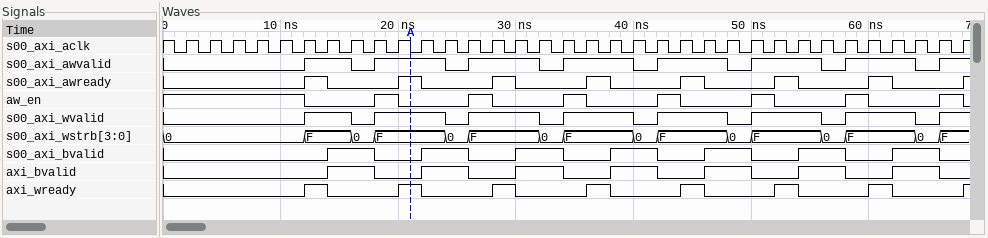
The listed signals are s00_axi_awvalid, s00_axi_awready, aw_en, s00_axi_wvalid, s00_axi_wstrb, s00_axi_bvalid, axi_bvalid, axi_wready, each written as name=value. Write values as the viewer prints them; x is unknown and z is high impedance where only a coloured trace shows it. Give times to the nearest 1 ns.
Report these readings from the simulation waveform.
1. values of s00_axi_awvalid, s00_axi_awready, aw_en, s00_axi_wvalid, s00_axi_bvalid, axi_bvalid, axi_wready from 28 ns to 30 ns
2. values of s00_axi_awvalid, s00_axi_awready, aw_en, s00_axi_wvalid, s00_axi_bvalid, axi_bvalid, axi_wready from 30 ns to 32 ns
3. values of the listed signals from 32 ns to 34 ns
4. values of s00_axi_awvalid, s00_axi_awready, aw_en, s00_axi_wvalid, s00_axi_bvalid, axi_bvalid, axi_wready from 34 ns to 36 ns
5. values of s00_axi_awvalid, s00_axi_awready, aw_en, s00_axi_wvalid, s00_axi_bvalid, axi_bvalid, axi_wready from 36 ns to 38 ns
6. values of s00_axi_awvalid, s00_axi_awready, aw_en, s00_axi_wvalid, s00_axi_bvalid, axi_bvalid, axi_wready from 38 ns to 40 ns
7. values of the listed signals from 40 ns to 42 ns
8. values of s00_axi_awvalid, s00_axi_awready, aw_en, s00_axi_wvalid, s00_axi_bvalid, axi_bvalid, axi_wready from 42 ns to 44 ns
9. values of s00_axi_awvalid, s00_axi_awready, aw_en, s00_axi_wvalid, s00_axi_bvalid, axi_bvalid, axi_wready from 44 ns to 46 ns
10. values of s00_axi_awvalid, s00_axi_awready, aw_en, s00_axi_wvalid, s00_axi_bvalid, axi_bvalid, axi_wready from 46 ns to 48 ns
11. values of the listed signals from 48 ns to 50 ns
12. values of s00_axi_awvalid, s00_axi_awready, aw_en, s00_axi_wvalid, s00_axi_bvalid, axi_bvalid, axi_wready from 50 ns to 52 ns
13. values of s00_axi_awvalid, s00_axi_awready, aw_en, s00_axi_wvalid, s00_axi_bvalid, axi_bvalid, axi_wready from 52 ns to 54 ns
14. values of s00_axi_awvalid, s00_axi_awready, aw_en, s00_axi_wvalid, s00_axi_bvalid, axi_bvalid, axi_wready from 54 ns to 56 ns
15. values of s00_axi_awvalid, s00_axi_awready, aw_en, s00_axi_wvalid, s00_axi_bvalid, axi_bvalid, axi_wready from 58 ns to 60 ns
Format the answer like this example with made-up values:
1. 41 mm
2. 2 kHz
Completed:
1. s00_axi_awvalid=1, s00_axi_awready=1, aw_en=0, s00_axi_wvalid=1, s00_axi_bvalid=0, axi_bvalid=0, axi_wready=1
2. s00_axi_awvalid=1, s00_axi_awready=0, aw_en=0, s00_axi_wvalid=1, s00_axi_bvalid=1, axi_bvalid=1, axi_wready=0
3. s00_axi_awvalid=0, s00_axi_awready=0, aw_en=0, s00_axi_wvalid=0, s00_axi_wstrb=0, s00_axi_bvalid=1, axi_bvalid=1, axi_wready=0
4. s00_axi_awvalid=1, s00_axi_awready=0, aw_en=1, s00_axi_wvalid=1, s00_axi_bvalid=0, axi_bvalid=0, axi_wready=0
5. s00_axi_awvalid=1, s00_axi_awready=1, aw_en=0, s00_axi_wvalid=1, s00_axi_bvalid=0, axi_bvalid=0, axi_wready=1
6. s00_axi_awvalid=1, s00_axi_awready=0, aw_en=0, s00_axi_wvalid=1, s00_axi_bvalid=1, axi_bvalid=1, axi_wready=0
7. s00_axi_awvalid=0, s00_axi_awready=0, aw_en=0, s00_axi_wvalid=0, s00_axi_wstrb=0, s00_axi_bvalid=1, axi_bvalid=1, axi_wready=0
8. s00_axi_awvalid=1, s00_axi_awready=0, aw_en=1, s00_axi_wvalid=1, s00_axi_bvalid=0, axi_bvalid=0, axi_wready=0
9. s00_axi_awvalid=1, s00_axi_awready=1, aw_en=0, s00_axi_wvalid=1, s00_axi_bvalid=0, axi_bvalid=0, axi_wready=1
10. s00_axi_awvalid=1, s00_axi_awready=0, aw_en=0, s00_axi_wvalid=1, s00_axi_bvalid=1, axi_bvalid=1, axi_wready=0
11. s00_axi_awvalid=0, s00_axi_awready=0, aw_en=0, s00_axi_wvalid=0, s00_axi_wstrb=0, s00_axi_bvalid=1, axi_bvalid=1, axi_wready=0
12. s00_axi_awvalid=1, s00_axi_awready=0, aw_en=1, s00_axi_wvalid=1, s00_axi_bvalid=0, axi_bvalid=0, axi_wready=0
13. s00_axi_awvalid=1, s00_axi_awready=1, aw_en=0, s00_axi_wvalid=1, s00_axi_bvalid=0, axi_bvalid=0, axi_wready=1
14. s00_axi_awvalid=1, s00_axi_awready=0, aw_en=0, s00_axi_wvalid=1, s00_axi_bvalid=1, axi_bvalid=1, axi_wready=0
15. s00_axi_awvalid=1, s00_axi_awready=0, aw_en=1, s00_axi_wvalid=1, s00_axi_bvalid=0, axi_bvalid=0, axi_wready=0
